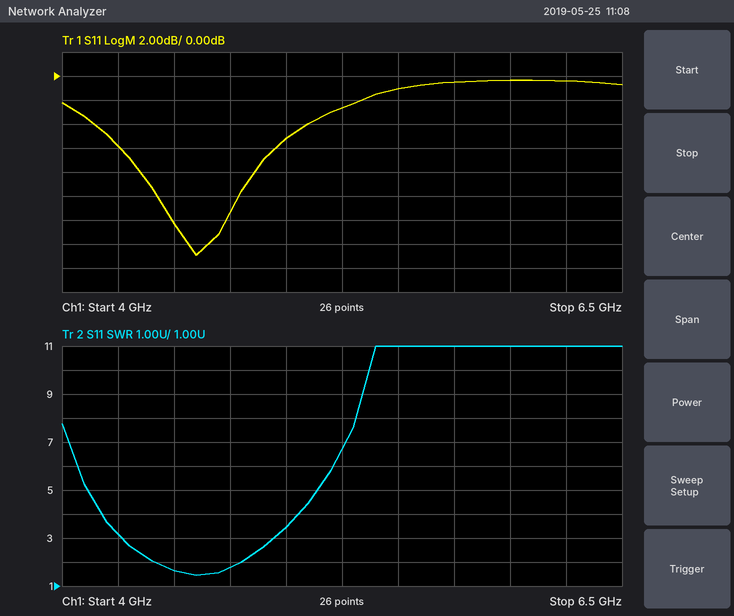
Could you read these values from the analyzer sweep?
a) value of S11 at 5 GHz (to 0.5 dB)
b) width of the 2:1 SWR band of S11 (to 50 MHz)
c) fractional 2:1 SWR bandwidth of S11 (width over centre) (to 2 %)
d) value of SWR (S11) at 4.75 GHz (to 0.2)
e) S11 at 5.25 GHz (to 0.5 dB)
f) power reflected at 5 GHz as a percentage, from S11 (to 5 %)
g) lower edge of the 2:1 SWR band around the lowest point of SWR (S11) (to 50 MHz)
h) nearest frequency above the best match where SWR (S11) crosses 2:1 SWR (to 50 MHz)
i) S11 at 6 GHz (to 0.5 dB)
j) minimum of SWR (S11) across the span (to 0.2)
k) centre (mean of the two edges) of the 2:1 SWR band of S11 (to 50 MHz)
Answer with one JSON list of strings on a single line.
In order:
["-5.0 dB", "400 MHz", "8 %", "1.8", "-2.5 dB", "30 %", "4.40 GHz", "4.80 GHz", "-0.5 dB", "1.4", "4.60 GHz"]
